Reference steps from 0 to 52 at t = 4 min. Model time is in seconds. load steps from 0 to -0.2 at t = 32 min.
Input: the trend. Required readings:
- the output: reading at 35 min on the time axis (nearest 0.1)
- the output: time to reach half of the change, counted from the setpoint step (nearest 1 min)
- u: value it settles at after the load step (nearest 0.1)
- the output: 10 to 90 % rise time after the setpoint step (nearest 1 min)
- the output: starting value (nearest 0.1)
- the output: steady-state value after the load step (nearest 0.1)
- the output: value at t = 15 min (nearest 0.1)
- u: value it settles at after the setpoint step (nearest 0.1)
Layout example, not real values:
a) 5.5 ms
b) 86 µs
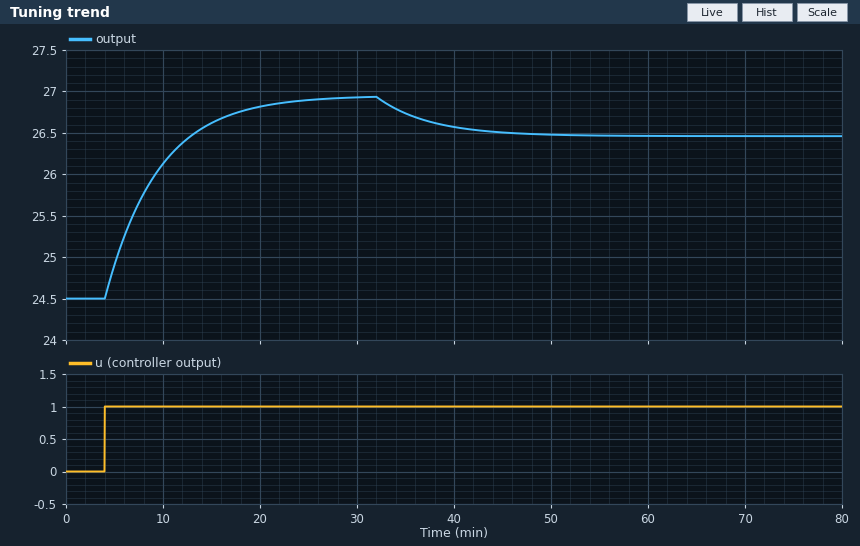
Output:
a) 26.7
b) 4 min
c) 1.0
d) 12 min
e) 24.5
f) 26.5
g) 26.6
h) 1.0
